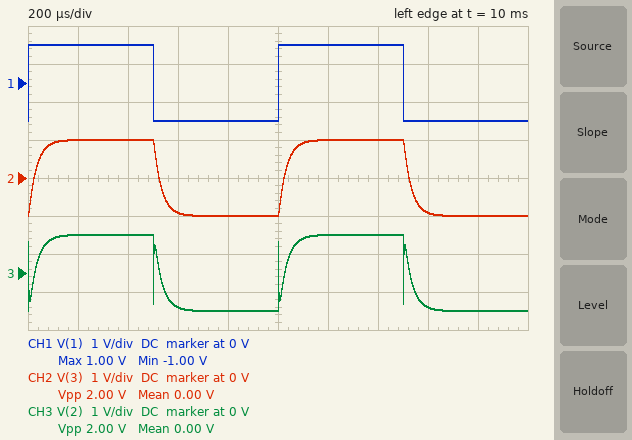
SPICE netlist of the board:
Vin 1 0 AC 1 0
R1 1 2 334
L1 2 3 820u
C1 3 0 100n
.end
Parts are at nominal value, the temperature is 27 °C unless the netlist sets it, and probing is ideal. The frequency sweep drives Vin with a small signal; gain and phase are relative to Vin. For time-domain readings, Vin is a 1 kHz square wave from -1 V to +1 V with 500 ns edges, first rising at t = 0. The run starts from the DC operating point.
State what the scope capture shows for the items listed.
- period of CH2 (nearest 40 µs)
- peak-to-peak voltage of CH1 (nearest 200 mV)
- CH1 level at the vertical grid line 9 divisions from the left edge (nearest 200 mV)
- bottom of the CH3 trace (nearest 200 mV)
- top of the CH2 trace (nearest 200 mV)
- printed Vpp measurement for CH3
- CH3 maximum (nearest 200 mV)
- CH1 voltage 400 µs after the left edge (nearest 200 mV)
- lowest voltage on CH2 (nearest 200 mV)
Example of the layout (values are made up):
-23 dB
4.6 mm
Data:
1.00 ms
2.0 V
-1.0 V
-1.0 V
1.0 V
2.00 V
1.0 V
1.0 V
-1.0 V
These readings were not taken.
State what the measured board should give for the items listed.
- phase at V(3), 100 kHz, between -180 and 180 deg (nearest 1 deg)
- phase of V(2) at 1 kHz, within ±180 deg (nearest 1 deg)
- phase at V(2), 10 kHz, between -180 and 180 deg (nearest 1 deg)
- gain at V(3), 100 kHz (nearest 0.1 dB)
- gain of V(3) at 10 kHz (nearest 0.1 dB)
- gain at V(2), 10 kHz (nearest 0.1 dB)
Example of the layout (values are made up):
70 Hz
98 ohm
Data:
-146 deg
-12 deg
-72 deg
-31.5 dB
-6.9 dB
-10.3 dB
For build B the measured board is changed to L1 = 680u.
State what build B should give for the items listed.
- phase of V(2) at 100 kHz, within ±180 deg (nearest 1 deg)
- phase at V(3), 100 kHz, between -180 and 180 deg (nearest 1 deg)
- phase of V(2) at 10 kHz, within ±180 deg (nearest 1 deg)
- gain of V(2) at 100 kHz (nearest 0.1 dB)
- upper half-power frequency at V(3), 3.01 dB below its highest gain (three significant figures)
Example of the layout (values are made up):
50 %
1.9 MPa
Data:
39 deg
-141 deg
-71 deg
-2.2 dB
5.07 kHz
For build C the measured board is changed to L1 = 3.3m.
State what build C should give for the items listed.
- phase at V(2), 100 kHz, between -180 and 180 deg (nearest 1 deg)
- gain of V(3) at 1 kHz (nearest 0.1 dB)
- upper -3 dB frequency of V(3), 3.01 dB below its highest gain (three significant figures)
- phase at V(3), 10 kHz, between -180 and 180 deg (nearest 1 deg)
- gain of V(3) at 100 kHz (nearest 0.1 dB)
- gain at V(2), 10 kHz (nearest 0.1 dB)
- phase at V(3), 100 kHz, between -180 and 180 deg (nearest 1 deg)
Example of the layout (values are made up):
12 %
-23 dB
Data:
9 deg
-0.1 dB
6.35 kHz
-98 deg
-42.3 dB
-16.9 dB
-171 deg
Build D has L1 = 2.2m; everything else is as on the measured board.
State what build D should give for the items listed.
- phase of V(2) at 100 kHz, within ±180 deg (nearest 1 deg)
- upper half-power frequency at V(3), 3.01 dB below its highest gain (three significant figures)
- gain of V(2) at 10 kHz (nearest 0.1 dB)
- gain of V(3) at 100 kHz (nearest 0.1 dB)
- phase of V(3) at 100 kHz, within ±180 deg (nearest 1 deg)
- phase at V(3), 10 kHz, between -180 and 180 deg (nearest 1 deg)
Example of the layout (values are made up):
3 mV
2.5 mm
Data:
14 deg
5.85 kHz
-24.1 dB
-38.9 dB
-166 deg
-86 deg
